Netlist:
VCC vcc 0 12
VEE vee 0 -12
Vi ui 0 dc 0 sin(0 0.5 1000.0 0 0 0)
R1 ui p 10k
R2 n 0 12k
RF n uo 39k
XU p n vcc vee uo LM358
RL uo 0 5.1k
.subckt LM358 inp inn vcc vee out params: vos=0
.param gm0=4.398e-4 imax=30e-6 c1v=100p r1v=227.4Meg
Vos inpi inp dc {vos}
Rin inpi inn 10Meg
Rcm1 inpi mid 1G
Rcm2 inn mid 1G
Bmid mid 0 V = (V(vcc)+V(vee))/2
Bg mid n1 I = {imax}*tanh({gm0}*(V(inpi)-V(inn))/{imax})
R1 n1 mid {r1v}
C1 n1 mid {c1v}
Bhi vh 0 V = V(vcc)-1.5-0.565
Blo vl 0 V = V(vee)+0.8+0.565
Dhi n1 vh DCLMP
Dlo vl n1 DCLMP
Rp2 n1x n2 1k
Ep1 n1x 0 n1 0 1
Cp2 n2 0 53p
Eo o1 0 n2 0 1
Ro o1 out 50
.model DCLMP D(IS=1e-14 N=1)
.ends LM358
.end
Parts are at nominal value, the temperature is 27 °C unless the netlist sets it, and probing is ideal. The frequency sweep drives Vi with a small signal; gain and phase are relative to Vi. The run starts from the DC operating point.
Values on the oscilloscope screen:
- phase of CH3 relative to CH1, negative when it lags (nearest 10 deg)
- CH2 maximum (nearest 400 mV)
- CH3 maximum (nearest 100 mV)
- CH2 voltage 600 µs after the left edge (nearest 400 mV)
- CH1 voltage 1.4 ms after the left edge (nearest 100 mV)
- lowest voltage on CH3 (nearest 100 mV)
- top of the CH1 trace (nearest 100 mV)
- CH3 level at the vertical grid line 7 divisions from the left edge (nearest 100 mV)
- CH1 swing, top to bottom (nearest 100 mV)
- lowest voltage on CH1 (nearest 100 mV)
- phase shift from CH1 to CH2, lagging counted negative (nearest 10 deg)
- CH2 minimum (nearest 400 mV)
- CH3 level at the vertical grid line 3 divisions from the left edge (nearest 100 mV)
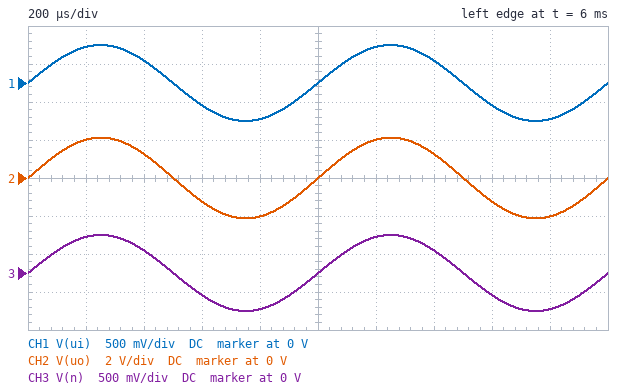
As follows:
0 deg
2.0 V
500 mV
-1.2 V
300 mV
-500 mV
500 mV
300 mV
1.0 V
-500 mV
0 deg
-2.0 V
-300 mV
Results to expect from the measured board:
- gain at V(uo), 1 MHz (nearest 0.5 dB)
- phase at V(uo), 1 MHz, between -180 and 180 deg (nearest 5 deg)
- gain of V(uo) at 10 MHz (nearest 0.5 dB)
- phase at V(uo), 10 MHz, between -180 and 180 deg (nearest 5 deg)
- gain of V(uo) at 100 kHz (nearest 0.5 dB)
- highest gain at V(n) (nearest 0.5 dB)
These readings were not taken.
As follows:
-3.5 dB
-100 deg
-34.0 dB
-165 deg
11.5 dB
0 dB
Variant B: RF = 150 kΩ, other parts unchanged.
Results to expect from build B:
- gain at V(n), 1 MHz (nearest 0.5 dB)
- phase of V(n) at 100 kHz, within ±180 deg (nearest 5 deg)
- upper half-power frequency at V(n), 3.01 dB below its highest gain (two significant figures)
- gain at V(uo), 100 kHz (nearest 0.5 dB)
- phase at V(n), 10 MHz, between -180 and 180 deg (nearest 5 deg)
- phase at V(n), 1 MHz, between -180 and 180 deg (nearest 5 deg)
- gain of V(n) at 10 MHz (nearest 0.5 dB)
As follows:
-26.0 dB
-65 deg
52 kHz
16.0 dB
-125 deg
-105 deg
-65.5 dB
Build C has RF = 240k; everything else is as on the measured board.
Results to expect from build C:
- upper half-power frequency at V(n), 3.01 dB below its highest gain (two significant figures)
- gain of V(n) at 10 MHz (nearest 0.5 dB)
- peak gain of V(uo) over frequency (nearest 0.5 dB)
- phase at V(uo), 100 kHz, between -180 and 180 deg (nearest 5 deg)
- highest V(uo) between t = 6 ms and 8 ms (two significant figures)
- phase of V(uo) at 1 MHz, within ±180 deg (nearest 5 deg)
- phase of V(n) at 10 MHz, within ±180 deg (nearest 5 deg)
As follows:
33 kHz
-69.0 dB
26.5 dB
-75 deg
10 V
-105 deg
-50 deg
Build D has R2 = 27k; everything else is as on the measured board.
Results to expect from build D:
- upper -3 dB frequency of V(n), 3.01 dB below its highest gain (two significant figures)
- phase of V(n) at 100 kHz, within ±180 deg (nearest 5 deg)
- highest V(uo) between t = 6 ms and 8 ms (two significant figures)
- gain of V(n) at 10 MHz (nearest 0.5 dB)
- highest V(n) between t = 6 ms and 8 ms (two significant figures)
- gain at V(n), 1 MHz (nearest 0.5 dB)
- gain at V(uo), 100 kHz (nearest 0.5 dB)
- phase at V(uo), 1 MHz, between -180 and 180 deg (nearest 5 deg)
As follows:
310 kHz
-20 deg
1.2 V
-43.5 dB
500 mV
-11.0 dB
7.5 dB
-95 deg
